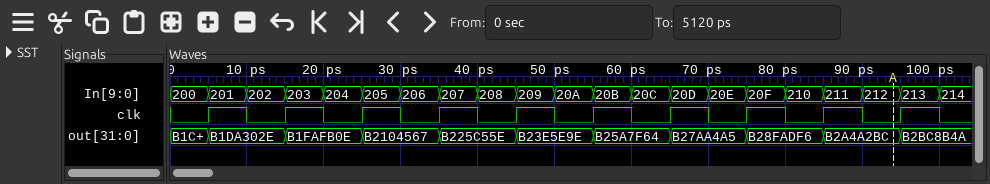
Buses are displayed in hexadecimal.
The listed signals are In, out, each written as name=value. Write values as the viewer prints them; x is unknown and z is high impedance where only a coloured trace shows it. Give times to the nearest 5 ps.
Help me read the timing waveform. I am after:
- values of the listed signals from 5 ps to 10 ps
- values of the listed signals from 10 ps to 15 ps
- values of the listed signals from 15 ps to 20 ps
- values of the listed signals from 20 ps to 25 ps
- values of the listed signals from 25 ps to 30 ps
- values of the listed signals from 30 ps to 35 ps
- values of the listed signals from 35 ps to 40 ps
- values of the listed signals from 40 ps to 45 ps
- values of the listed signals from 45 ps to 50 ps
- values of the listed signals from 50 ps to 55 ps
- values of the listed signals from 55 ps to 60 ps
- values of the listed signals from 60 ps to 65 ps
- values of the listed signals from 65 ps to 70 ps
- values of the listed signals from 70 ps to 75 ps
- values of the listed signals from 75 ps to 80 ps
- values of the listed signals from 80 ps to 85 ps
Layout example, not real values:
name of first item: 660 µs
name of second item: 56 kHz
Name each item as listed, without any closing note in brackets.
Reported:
values of the listed signals from 5 ps to 10 ps: In=201, out=B1DA302E
values of the listed signals from 10 ps to 15 ps: In=202, out=B1DA302E
values of the listed signals from 15 ps to 20 ps: In=203, out=B1FAFB0E
values of the listed signals from 20 ps to 25 ps: In=204, out=B1FAFB0E
values of the listed signals from 25 ps to 30 ps: In=205, out=B2104567
values of the listed signals from 30 ps to 35 ps: In=206, out=B2104567
values of the listed signals from 35 ps to 40 ps: In=207, out=B225C55E
values of the listed signals from 40 ps to 45 ps: In=208, out=B225C55E
values of the listed signals from 45 ps to 50 ps: In=209, out=B23E5E9E
values of the listed signals from 50 ps to 55 ps: In=20A, out=B23E5E9E
values of the listed signals from 55 ps to 60 ps: In=20B, out=B25A7F64
values of the listed signals from 60 ps to 65 ps: In=20C, out=B25A7F64
values of the listed signals from 65 ps to 70 ps: In=20D, out=B27AA4A5
values of the listed signals from 70 ps to 75 ps: In=20E, out=B27AA4A5
values of the listed signals from 75 ps to 80 ps: In=20F, out=B28FADF6
values of the listed signals from 80 ps to 85 ps: In=210, out=B28FADF6
